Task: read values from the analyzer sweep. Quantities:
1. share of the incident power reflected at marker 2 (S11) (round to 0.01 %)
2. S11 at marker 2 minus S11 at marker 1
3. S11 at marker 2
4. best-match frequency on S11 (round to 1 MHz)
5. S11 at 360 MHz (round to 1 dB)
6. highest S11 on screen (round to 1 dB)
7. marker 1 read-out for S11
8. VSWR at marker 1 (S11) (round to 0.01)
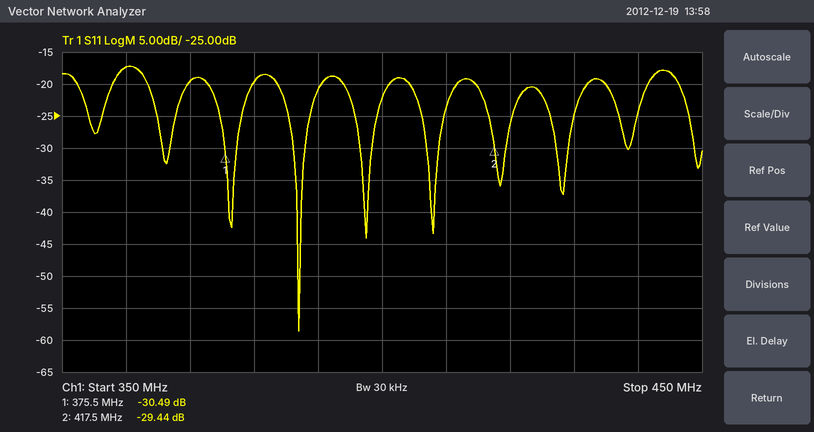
0.11 %
1.05 dB
-29.44 dB
387 MHz
-17 dB
-17 dB
-30.49 dB
1.06
